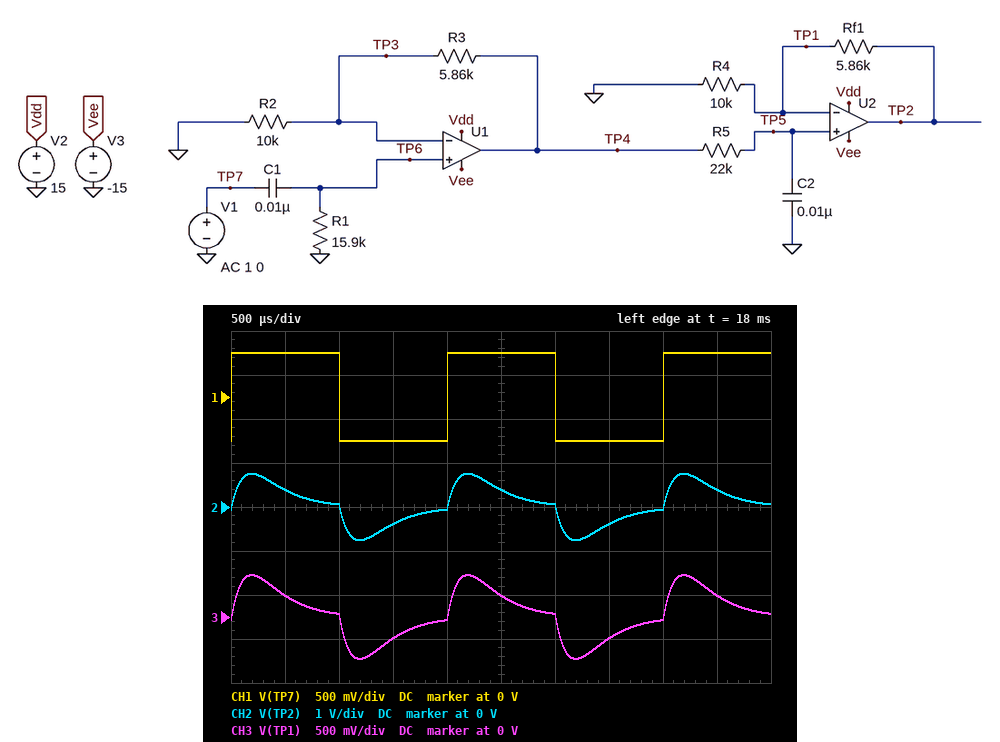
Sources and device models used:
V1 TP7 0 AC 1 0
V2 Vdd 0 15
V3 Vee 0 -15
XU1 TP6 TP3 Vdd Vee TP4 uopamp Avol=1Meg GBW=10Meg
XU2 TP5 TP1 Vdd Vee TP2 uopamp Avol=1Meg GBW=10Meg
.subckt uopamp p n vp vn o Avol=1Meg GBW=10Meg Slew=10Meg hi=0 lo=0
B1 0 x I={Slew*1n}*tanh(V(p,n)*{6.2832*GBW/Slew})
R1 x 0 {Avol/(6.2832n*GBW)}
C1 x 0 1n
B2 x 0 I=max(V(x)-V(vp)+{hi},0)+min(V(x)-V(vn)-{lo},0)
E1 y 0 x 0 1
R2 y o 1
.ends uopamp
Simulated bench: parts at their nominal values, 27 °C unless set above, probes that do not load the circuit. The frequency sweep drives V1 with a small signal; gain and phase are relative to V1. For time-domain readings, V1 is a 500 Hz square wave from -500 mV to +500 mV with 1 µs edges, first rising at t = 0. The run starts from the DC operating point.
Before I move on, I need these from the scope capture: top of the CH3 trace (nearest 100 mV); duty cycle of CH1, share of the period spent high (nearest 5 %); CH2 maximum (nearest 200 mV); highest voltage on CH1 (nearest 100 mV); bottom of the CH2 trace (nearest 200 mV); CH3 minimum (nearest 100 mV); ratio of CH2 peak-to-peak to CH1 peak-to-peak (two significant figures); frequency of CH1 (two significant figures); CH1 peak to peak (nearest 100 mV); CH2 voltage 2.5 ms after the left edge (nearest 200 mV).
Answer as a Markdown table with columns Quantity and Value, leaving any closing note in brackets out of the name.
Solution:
| Quantity | Value |
|---|---|
| top of the CH3 trace | 500 mV |
| duty cycle of CH1, share of the period spent high | 50 % |
| CH2 maximum | 800 mV |
| highest voltage on CH1 | 500 mV |
| bottom of the CH2 trace | -800 mV |
| CH3 minimum | -500 mV |
| ratio of CH2 peak-to-peak to CH1 peak-to-peak | 1.5 |
| frequency of CH1 | 500 Hz |
| CH1 peak to peak | 1.0 V |
| CH2 voltage 2.5 ms after the left edge | 400 mV |
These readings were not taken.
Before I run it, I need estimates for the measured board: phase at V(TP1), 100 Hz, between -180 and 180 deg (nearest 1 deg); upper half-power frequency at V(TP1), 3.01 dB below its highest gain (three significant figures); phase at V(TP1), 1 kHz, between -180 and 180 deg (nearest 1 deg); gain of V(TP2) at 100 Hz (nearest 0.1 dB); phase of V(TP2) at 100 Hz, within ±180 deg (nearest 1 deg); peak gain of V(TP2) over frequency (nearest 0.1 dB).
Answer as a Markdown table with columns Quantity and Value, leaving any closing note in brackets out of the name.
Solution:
| Quantity | Value |
|---|---|
| phase at V(TP1), 100 Hz, between -180 and 180 deg | 76 deg |
| upper half-power frequency at V(TP1), 3.01 dB below its highest gain | 2.07 kHz |
| phase at V(TP1), 1 kHz, between -180 and 180 deg | -9 deg |
| gain of V(TP2) at 100 Hz | -12.1 dB |
| phase of V(TP2) at 100 Hz, within ±180 deg | 76 deg |
| peak gain of V(TP2) over frequency | 0.5 dB |
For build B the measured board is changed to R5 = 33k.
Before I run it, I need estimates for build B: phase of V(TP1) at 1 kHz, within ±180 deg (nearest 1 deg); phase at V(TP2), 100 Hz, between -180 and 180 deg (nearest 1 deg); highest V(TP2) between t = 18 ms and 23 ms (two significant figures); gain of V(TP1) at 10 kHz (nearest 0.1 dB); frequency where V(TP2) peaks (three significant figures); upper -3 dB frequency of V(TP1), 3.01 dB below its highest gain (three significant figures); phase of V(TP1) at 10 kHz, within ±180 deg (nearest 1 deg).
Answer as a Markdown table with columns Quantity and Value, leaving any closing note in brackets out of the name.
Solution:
| Quantity | Value |
|---|---|
| phase of V(TP1) at 1 kHz, within ±180 deg | -19 deg |
| phase at V(TP2), 100 Hz, between -180 and 180 deg | 73 deg |
| highest V(TP2) between t = 18 ms and 23 ms | 560 mV |
| gain of V(TP1) at 10 kHz | -22.4 dB |
| frequency where V(TP2) peaks | 695 Hz |
| upper -3 dB frequency of V(TP1), 3.01 dB below its highest gain | 1.76 kHz |
| phase of V(TP1) at 10 kHz, within ±180 deg | -82 deg |
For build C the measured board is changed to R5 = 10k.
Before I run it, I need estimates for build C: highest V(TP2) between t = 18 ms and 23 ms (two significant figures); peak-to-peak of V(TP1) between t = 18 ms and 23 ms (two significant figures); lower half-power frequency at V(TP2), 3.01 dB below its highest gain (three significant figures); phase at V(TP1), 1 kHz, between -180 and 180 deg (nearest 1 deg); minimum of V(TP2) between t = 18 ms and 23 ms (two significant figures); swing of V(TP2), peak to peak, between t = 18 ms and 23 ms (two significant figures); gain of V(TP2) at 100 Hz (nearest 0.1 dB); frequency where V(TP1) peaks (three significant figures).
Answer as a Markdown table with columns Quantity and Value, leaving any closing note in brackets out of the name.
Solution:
| Quantity | Value |
|---|---|
| highest V(TP2) between t = 18 ms and 23 ms | 1.1 V |
| peak-to-peak of V(TP1) between t = 18 ms and 23 ms | 1.4 V |
| lower half-power frequency at V(TP2), 3.01 dB below its highest gain | 513 Hz |
| phase at V(TP1), 1 kHz, between -180 and 180 deg | 13 deg |
| minimum of V(TP2) between t = 18 ms and 23 ms | -1.1 V |
| swing of V(TP2), peak to peak, between t = 18 ms and 23 ms | 2.3 V |
| gain of V(TP2) at 100 Hz | -12.1 dB |
| frequency where V(TP1) peaks | 1.26 kHz |
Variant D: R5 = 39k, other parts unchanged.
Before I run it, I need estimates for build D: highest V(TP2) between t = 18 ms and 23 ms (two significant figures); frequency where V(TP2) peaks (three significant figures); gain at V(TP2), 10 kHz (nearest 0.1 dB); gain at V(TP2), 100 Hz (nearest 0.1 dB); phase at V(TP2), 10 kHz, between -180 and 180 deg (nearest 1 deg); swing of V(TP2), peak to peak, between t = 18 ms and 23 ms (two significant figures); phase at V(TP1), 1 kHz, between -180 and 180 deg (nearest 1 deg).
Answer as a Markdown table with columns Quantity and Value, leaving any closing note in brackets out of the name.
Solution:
| Quantity | Value |
|---|---|
| highest V(TP2) between t = 18 ms and 23 ms | 490 mV |
| frequency where V(TP2) peaks | 639 Hz |
| gain at V(TP2), 10 kHz | -19.8 dB |
| gain at V(TP2), 100 Hz | -12.3 dB |
| phase at V(TP2), 10 kHz, between -180 and 180 deg | -82 deg |
| swing of V(TP2), peak to peak, between t = 18 ms and 23 ms | 980 mV |
| phase at V(TP1), 1 kHz, between -180 and 180 deg | -23 deg |
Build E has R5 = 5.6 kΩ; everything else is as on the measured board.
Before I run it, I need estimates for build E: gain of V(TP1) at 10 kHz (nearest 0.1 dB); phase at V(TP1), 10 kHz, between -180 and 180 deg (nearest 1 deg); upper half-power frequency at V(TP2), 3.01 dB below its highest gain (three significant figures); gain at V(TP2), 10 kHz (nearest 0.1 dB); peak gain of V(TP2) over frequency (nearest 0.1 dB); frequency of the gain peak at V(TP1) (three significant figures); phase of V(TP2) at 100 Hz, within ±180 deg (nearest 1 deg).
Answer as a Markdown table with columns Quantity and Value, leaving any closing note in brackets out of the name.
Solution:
| Quantity | Value |
|---|---|
| gain of V(TP1) at 10 kHz | -7.3 dB |
| phase at V(TP1), 10 kHz, between -180 and 180 deg | -69 deg |
| upper half-power frequency at V(TP2), 3.01 dB below its highest gain | 4.48 kHz |
| gain at V(TP2), 10 kHz | -3.3 dB |
| peak gain of V(TP2) over frequency | 5.4 dB |
| frequency of the gain peak at V(TP1) | 1.69 kHz |
| phase of V(TP2) at 100 Hz, within ±180 deg | 82 deg |
